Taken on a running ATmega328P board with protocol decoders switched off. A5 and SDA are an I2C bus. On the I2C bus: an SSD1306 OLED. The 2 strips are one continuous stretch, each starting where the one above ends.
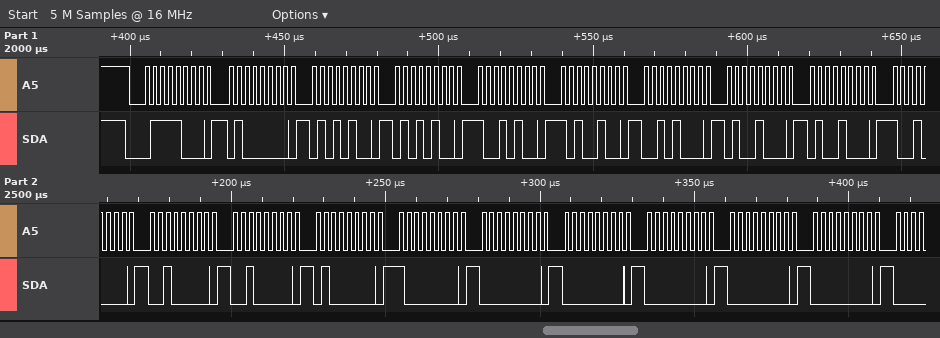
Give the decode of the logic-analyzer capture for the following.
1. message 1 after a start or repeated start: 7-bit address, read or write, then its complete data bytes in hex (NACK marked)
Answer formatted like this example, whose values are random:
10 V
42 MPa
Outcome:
0x3C write: 40 54 54 94 A4 28 48 48 90 20 20 40 80 00 00 00 00 00
